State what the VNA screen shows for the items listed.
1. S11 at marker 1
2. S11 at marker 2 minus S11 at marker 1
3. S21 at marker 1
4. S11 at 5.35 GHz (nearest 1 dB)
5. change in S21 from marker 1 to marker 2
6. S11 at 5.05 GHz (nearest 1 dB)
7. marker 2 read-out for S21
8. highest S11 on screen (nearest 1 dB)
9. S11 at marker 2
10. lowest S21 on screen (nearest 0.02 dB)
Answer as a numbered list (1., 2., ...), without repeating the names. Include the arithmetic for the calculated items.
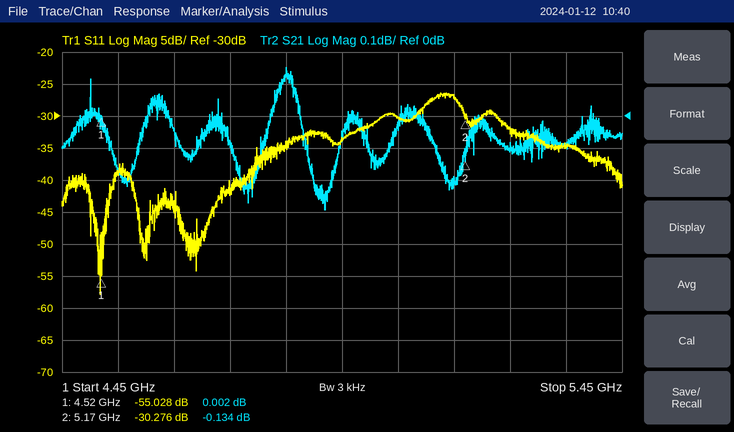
1. -55.028 dB
2. -30.276 − (-55.028) = 24.752 dB
3. 0.002 dB
4. -35 dB
5. -0.134 − (0.002) = -0.136 dB
6. -30 dB
7. -0.134 dB
8. -26 dB
9. -30.276 dB
10. -0.30 dB
